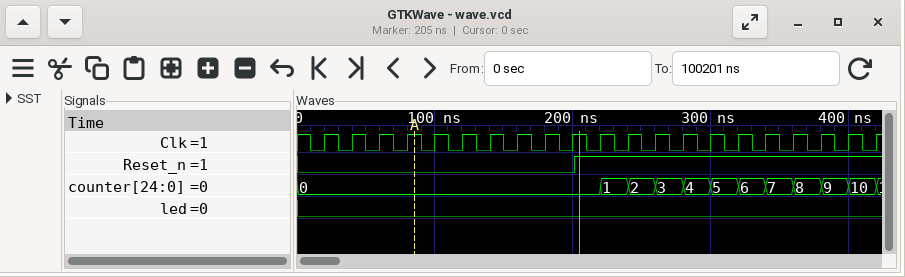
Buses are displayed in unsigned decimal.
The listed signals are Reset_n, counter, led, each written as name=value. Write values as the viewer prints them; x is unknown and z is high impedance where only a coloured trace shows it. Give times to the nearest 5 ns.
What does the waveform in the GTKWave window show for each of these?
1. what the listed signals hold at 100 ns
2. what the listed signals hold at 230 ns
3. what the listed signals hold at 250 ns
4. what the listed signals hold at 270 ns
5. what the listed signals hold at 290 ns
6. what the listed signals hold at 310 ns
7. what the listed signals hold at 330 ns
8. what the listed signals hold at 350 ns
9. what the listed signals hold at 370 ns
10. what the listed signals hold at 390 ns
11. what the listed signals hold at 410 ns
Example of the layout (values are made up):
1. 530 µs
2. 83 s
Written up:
1. Reset_n=0, counter=0, led=0
2. Reset_n=1, counter=1, led=0
3. Reset_n=1, counter=2, led=0
4. Reset_n=1, counter=3, led=0
5. Reset_n=1, counter=4, led=0
6. Reset_n=1, counter=5, led=0
7. Reset_n=1, counter=6, led=0
8. Reset_n=1, counter=7, led=0
9. Reset_n=1, counter=8, led=0
10. Reset_n=1, counter=9, led=0
11. Reset_n=1, counter=10, led=0
